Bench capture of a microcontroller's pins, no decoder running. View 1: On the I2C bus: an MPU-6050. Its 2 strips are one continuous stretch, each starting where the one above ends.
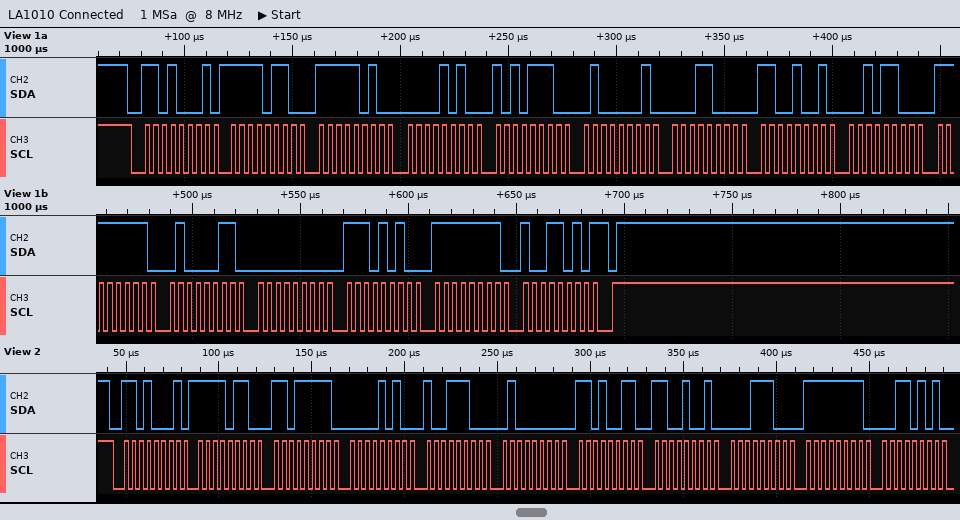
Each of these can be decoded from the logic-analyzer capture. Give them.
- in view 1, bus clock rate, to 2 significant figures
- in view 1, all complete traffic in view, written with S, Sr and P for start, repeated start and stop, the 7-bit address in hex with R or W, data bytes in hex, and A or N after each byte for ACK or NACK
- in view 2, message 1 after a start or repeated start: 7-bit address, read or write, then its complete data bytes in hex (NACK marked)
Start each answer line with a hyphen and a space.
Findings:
- 250 kHz
- S 68R A F6 A FA A 0A A AE A 41 A 18 A C9 A 2C A FF A 43 A 00 A EA A FF A 9A N P
- 0x68 read: F6 DF 0A 9C 40 D3 C9 1C FF 35
